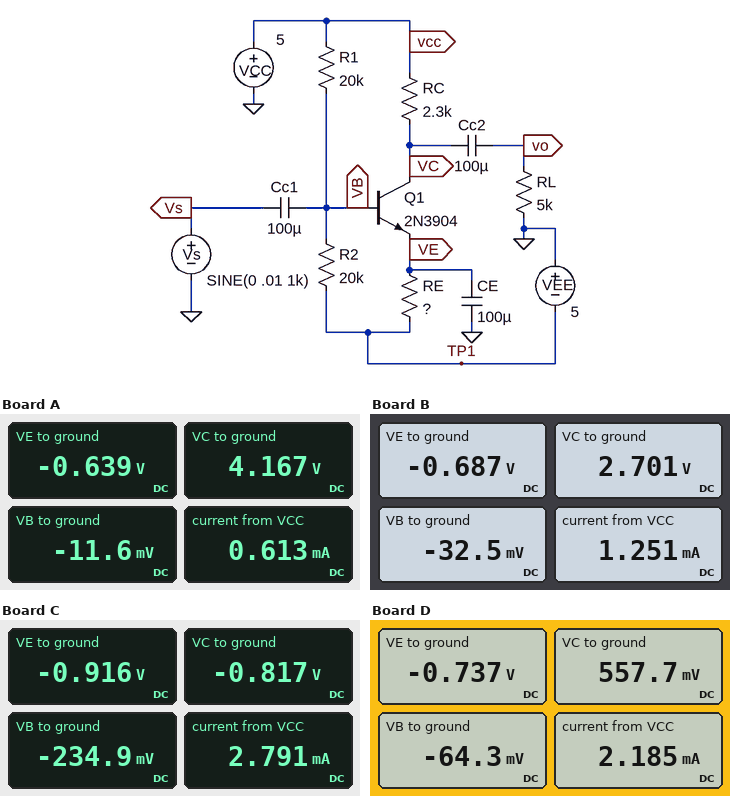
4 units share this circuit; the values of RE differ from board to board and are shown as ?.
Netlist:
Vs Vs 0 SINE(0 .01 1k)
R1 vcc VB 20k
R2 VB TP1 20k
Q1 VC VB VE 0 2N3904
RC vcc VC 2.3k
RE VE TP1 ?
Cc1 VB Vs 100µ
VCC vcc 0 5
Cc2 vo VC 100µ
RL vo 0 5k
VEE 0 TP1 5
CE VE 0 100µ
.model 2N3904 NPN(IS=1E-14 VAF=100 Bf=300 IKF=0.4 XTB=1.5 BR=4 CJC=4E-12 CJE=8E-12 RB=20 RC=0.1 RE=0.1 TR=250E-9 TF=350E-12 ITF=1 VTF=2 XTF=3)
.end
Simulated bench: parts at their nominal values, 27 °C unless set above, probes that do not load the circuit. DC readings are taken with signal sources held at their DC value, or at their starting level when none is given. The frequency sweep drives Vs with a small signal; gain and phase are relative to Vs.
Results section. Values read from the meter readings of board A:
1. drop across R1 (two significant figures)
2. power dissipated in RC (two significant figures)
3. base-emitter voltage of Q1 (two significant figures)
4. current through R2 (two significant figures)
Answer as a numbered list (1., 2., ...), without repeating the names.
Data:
1. 5.0 V
2. 300 µW
3. 630 mV
4. 250 µA
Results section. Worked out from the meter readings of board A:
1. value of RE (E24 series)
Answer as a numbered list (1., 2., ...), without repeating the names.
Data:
1. 12 kΩ
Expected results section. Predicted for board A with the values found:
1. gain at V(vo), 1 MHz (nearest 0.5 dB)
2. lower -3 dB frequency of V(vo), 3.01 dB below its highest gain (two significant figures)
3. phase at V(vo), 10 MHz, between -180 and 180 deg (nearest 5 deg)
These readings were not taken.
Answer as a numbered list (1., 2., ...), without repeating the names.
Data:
1. 27.0 dB
2. 22 Hz
3. 165 deg
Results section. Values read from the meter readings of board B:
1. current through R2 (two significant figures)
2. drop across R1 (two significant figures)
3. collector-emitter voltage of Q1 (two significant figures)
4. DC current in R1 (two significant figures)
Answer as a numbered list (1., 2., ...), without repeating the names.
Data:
1. 250 µA
2. 5.0 V
3. 3.4 V
4. 250 µA
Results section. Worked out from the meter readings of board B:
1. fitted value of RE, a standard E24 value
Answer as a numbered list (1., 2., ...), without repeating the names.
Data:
1. 4.3 kΩ
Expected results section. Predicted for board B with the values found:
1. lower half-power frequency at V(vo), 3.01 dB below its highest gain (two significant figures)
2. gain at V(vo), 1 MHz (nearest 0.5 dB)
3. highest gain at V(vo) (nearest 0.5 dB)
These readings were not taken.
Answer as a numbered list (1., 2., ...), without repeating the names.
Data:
1. 61 Hz
2. 35.5 dB
3. 35.5 dB
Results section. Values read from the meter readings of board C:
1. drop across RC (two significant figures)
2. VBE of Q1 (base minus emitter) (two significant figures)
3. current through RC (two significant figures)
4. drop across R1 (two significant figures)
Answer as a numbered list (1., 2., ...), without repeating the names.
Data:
1. 5.8 V
2. 680 mV
3. 2.5 mA
4. 5.2 V
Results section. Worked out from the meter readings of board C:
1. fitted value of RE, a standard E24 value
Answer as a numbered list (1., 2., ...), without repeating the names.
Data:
1. 1.6 kΩ
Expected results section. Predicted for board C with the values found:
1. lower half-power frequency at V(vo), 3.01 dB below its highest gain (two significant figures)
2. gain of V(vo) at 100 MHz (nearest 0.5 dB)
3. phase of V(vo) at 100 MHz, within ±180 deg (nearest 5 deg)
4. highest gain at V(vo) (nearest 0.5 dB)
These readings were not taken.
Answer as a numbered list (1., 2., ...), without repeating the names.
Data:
1. 62 Hz
2. -9.5 dB
3. 5 deg
4. 26.5 dB
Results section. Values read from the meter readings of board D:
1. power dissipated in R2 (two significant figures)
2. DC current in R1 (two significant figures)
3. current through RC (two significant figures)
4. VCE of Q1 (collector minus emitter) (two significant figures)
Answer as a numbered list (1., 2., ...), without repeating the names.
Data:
1. 1.2 mW
2. 250 µA
3. 1.9 mA
4. 1.3 V
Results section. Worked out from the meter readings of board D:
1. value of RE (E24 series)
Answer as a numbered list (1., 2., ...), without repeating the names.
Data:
1. 2.2 kΩ
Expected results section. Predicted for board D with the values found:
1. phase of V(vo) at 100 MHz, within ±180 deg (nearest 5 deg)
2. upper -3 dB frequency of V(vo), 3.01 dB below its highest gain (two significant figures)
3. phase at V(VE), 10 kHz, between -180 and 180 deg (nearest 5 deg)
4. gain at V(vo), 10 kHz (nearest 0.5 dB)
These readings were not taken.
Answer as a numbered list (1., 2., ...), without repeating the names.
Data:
1. 85 deg
2. 12 MHz
3. -90 deg
4. 41.0 dB
